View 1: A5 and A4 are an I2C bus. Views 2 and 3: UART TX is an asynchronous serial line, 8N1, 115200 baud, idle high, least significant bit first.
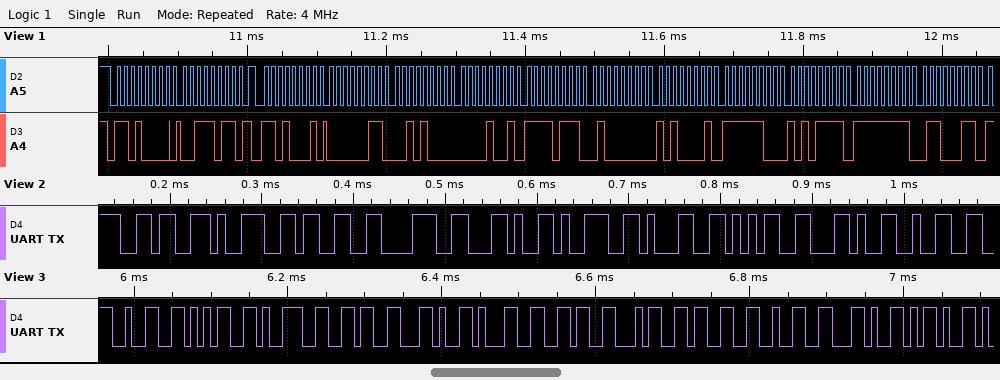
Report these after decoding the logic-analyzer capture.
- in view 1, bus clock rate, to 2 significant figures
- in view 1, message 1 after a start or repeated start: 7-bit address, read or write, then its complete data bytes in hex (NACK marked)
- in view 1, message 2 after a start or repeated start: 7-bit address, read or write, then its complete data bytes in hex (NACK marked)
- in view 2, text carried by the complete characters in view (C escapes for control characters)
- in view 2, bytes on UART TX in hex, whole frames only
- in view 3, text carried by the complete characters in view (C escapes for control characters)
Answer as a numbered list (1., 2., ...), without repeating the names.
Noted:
1. 100 kHz
2. 0x68 write: 3B
3. 0x68 read: 03 28 09 F7 40 A1 FC AF FF 63
4. "6938,915,2"
5. 36 39 33 38 2C 39 31 35 2C 32
6. "2596,16432,-"
